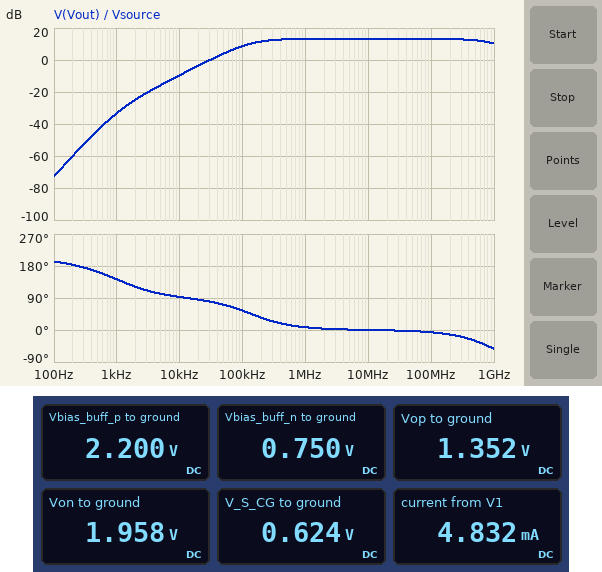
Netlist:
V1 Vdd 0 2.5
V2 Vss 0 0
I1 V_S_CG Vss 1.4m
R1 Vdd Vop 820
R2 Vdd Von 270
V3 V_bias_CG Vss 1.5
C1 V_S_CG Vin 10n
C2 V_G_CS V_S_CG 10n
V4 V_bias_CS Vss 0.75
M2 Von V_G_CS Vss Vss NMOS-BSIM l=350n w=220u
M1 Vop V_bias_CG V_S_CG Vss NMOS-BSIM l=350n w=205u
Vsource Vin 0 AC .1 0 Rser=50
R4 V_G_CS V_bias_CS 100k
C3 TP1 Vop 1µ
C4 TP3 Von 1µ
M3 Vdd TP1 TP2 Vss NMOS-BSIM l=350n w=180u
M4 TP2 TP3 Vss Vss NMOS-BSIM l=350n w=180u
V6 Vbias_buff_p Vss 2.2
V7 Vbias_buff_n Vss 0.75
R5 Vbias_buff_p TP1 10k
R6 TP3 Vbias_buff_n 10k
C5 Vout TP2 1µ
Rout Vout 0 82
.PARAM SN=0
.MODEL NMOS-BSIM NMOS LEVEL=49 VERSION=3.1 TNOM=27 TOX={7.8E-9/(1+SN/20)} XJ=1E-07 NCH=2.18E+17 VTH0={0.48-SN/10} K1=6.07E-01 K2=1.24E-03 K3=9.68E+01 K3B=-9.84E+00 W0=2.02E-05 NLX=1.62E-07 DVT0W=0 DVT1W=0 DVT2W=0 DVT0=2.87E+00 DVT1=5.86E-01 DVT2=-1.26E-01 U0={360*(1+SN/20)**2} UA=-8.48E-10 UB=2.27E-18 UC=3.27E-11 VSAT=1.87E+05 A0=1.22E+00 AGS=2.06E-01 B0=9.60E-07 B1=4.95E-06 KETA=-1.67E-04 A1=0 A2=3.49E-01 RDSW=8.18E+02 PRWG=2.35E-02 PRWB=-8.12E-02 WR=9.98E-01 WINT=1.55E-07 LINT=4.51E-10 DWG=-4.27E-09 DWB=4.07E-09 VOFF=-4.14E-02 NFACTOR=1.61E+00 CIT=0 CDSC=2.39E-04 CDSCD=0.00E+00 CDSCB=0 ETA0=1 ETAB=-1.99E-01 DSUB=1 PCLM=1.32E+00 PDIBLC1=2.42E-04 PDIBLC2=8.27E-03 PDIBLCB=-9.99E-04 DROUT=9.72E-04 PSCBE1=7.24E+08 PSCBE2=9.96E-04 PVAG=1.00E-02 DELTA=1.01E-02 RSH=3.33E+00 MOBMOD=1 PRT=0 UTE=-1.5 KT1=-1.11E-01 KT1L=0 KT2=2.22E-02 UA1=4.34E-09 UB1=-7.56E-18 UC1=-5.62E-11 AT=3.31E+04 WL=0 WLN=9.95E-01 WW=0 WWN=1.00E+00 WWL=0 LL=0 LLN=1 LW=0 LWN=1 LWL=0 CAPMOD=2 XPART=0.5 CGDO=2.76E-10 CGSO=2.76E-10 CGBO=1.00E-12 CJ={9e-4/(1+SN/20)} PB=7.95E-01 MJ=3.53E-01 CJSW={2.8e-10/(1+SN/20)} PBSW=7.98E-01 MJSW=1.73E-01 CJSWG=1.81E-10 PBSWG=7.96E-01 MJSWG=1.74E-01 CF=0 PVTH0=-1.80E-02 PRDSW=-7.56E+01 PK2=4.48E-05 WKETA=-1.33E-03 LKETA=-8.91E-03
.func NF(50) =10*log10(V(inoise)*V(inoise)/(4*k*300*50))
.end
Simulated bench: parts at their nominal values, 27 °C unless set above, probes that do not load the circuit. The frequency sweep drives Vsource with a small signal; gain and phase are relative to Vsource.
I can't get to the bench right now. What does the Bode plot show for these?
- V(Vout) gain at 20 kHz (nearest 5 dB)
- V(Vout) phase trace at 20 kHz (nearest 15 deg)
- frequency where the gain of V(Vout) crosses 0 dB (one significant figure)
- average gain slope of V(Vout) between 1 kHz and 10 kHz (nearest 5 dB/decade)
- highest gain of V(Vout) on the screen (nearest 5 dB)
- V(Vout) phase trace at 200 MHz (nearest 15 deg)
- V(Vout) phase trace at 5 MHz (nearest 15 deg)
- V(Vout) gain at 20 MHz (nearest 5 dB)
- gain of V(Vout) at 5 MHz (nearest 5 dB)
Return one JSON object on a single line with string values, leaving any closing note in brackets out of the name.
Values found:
{"V(Vout) gain at 20 kHz": "-5 dB", "V(Vout) phase trace at 20 kHz": "90 deg", "frequency where the gain of V(Vout) crosses 0 dB": "30 kHz", "average gain slope of V(Vout) between 1 kHz and 10 kHz": "25 dB/decade", "highest gain of V(Vout) on the screen": "15 dB", "V(Vout) phase trace at 200 MHz": "-15 deg", "V(Vout) phase trace at 5 MHz": "0 deg", "V(Vout) gain at 20 MHz": "15 dB", "gain of V(Vout) at 5 MHz": "15 dB"}
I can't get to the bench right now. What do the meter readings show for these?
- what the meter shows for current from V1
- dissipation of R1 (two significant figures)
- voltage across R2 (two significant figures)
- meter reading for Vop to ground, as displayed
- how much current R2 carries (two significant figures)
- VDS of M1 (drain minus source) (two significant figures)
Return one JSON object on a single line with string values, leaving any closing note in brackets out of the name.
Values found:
{"what the meter shows for current from V1": "4.832 mA", "dissipation of R1": "1.6 mW", "voltage across R2": "540 mV", "meter reading for Vop to ground, as displayed": "1.352 V", "how much current R2 carries": "2.0 mA", "VDS of M1 (drain minus source)": "730 mV"}
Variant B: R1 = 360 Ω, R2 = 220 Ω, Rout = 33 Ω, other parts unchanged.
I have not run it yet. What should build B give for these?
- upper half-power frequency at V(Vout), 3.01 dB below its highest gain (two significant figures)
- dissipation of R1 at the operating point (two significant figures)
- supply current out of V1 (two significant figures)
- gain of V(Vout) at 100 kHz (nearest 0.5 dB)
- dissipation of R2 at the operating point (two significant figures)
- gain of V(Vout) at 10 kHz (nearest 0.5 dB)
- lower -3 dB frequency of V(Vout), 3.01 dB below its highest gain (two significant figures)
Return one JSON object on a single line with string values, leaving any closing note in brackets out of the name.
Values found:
{"upper half-power frequency at V(Vout), 3.01 dB below its highest gain": "1.6 GHz", "dissipation of R1 at the operating point": "710 µW", "supply current out of V1": "4.9 mA", "gain of V(Vout) at 100 kHz": "-0.5 dB", "dissipation of R2 at the operating point": "920 µW", "gain of V(Vout) at 10 kHz": "-19.0 dB", "lower -3 dB frequency of V(Vout), 3.01 dB below its highest gain": "150 kHz"}
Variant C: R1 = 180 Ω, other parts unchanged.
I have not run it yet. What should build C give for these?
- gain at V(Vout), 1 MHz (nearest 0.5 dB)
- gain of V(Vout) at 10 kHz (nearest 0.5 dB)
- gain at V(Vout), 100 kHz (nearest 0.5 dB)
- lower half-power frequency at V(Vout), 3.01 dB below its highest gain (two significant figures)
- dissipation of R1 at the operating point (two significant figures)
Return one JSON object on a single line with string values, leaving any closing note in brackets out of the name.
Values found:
{"gain at V(Vout), 1 MHz": "6.0 dB", "gain of V(Vout) at 10 kHz": "-17.5 dB", "gain at V(Vout), 100 kHz": "1.0 dB", "lower half-power frequency at V(Vout), 3.01 dB below its highest gain": "150 kHz", "dissipation of R1 at the operating point": "350 µW"}
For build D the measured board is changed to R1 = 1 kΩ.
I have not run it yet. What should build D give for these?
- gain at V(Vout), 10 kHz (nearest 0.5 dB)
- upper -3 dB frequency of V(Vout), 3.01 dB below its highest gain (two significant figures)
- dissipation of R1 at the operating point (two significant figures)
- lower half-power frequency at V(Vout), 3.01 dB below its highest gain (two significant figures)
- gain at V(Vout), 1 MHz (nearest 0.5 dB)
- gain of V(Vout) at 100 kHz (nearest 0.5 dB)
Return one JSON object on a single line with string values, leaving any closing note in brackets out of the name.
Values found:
{"gain at V(Vout), 10 kHz": "-8.0 dB", "upper -3 dB frequency of V(Vout), 3.01 dB below its highest gain": "900 MHz", "dissipation of R1 at the operating point": "2.0 mW", "lower half-power frequency at V(Vout), 3.01 dB below its highest gain": "130 kHz", "gain at V(Vout), 1 MHz": "14.0 dB", "gain of V(Vout) at 100 kHz": "10.0 dB"}
